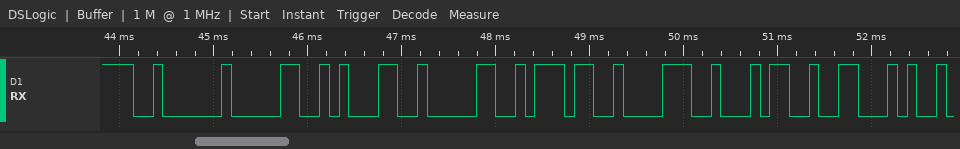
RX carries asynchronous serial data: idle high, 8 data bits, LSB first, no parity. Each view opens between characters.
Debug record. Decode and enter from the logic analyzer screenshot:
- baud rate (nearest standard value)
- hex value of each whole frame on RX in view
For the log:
9600 baud
02, 30, 31, 30, 37, 38, 34, 46
